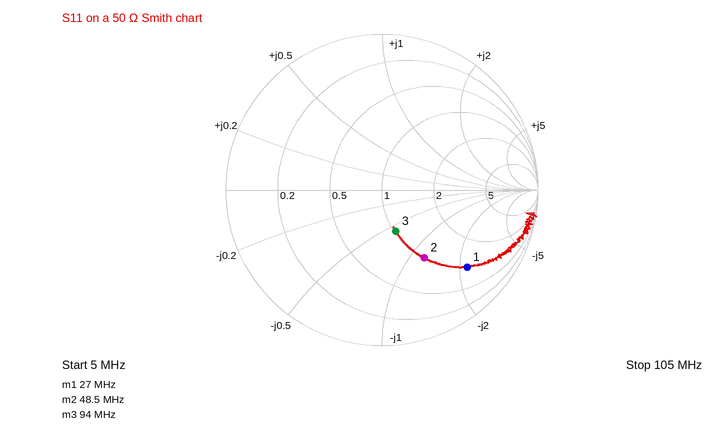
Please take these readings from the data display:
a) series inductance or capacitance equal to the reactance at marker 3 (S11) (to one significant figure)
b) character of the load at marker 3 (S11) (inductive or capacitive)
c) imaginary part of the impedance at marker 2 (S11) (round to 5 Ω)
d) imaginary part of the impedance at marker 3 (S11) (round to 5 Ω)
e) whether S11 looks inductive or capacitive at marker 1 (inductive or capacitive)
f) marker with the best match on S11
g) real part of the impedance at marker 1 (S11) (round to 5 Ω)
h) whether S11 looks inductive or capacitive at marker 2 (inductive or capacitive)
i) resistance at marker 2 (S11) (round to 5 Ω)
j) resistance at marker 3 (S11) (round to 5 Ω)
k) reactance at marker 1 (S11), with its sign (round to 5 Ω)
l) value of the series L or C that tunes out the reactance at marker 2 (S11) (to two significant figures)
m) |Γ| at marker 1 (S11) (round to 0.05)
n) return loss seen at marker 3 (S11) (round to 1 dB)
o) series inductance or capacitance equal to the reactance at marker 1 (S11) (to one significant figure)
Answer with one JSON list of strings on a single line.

["60 pF", "capacitive", "-60 Ω", "-30 Ω", "capacitive", "marker 3", "50 Ω", "capacitive", "50 Ω", "50 Ω", "-110 Ω", "200 nH", "0.75", "11 dB", "50 pF"]
